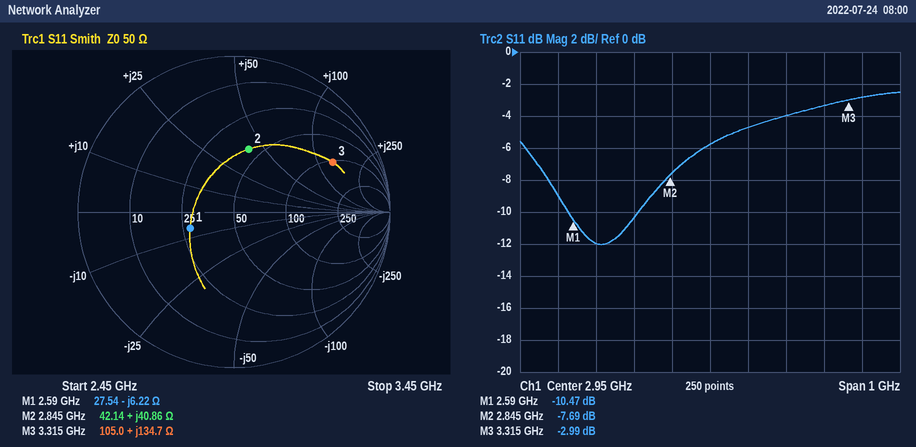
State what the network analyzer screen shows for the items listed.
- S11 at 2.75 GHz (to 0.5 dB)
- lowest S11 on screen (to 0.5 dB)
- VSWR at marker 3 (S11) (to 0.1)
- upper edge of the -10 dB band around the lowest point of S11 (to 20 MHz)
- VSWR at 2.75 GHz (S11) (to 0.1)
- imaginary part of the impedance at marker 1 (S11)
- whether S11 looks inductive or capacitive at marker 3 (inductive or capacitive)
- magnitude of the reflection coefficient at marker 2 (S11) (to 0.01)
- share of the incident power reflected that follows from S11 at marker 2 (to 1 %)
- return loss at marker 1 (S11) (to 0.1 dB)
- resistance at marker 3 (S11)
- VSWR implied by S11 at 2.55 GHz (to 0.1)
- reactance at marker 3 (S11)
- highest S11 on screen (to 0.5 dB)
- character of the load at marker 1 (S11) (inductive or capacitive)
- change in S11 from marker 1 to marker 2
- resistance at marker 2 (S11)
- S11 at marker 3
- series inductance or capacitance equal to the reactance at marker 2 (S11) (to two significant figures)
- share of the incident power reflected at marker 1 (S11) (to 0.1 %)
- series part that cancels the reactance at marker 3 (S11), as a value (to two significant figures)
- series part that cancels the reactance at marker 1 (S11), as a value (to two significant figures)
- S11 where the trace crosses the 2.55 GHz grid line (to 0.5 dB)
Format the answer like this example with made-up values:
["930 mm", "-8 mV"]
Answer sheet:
["-10.5 dB", "-12.0 dB", "5.9", "2.76 GHz", "1.9", "-6.22 Ω", "inductive", "0.41", "17 %", "10.5 dB", "105.0 Ω", "2.1", "+134.7 Ω", "-2.5 dB", "capacitive", "2.78 dB", "42.14 Ω", "-2.99 dB", "2.3 nH", "9.0 %", "360 fF", "380 pH", "-9.0 dB"]
